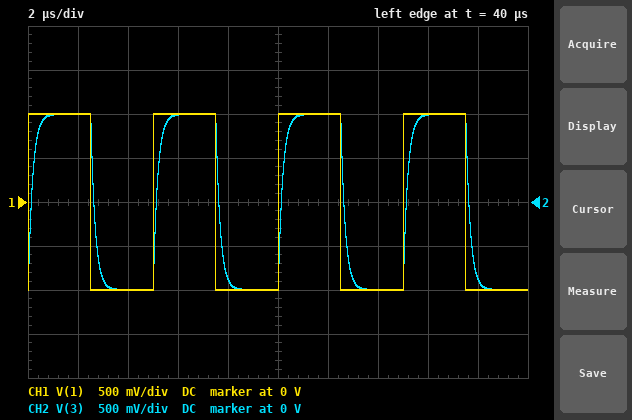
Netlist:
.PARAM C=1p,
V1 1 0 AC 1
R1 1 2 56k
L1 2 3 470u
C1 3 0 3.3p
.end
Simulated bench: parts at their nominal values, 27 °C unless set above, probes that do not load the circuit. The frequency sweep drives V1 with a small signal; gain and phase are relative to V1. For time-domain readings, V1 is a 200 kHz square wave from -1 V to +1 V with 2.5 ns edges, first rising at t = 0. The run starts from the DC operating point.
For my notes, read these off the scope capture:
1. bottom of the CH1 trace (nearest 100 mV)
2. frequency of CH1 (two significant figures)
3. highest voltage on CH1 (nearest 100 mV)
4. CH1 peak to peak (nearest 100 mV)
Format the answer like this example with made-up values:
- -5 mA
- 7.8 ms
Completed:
- -1.0 V
- 200 kHz
- 1.0 V
- 2.0 V
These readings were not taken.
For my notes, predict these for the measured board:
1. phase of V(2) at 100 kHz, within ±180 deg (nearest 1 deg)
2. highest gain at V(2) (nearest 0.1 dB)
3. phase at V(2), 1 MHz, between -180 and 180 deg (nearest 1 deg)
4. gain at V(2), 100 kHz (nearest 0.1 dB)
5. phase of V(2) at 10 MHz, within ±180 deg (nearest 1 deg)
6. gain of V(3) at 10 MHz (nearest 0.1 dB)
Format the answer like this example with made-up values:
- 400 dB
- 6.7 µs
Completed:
- -7 deg
- 0 dB
- -51 deg
- -0.1 dB
- 66 deg
- -22.1 dB
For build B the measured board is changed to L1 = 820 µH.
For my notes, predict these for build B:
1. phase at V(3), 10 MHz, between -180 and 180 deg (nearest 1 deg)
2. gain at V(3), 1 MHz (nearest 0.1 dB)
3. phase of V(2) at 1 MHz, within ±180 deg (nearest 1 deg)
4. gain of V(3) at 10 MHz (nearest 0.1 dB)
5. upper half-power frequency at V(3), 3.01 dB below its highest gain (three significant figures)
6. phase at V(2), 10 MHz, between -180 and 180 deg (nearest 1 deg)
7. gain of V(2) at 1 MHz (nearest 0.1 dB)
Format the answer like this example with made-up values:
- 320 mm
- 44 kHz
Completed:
- -130 deg
- -3.3 dB
- -52 deg
- -23.6 dB
- 935 kHz
- 50 deg
- -4.3 dB
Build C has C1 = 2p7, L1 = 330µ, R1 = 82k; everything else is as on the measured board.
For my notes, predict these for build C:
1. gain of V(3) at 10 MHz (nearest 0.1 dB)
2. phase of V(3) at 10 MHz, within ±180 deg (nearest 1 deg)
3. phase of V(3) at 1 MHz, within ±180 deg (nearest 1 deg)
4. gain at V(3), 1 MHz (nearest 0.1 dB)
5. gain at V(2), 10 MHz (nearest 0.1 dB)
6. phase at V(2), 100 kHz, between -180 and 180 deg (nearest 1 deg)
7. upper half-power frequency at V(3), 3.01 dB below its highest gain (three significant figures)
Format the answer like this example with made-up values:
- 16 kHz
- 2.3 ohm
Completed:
- -23.0 dB
- -100 deg
- -55 deg
- -4.6 dB
- -15.0 dB
- -8 deg
- 732 kHz
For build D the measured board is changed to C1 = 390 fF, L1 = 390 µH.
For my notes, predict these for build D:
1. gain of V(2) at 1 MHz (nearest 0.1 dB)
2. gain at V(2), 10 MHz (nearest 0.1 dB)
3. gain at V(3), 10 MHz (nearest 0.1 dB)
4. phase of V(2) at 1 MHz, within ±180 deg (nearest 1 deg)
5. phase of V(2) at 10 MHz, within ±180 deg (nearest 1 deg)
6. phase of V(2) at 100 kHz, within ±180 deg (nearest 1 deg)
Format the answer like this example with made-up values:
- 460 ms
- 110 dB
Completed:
- -0.1 dB
- -11.1 dB
- -3.1 dB
- -8 deg
- -74 deg
- -1 deg
